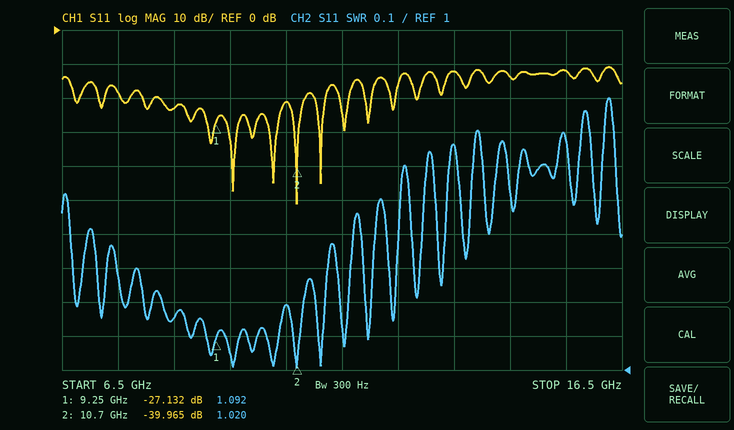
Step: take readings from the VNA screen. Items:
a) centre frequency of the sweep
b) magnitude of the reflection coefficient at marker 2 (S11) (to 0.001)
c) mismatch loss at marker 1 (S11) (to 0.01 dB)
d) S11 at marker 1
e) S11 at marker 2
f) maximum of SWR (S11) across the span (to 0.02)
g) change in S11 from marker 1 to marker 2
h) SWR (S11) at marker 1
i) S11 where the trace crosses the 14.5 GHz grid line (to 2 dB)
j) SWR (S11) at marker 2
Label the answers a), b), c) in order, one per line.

a) 11.5 GHz
b) 0.010
c) 0.01 dB
d) -27.132 dB
e) -39.965 dB
f) 1.80
g) -12.833 dB
h) 1.092
i) -14 dB
j) 1.020
